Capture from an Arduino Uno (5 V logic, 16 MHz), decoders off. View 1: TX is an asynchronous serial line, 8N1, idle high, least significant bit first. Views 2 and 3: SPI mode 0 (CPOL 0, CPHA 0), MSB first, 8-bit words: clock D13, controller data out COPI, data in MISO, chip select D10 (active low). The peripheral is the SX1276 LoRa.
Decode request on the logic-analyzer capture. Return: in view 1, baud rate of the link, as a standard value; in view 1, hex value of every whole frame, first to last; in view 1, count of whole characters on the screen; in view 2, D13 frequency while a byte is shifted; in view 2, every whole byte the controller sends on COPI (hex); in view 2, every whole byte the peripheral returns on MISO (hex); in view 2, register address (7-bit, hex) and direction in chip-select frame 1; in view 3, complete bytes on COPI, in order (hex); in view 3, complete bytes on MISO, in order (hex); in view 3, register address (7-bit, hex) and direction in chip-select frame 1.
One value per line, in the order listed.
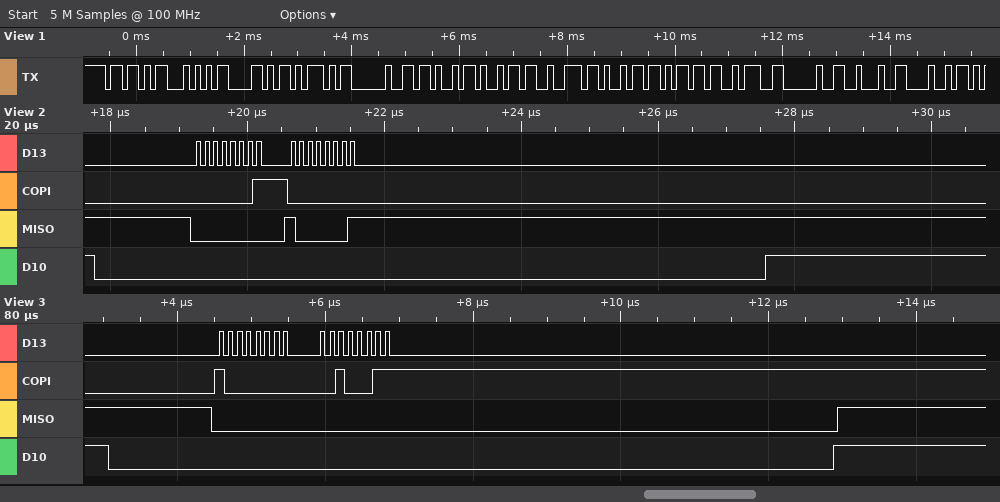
9600 baud
5B 54 58 5D 20 4B 69 72 69 6D 3A 20 22 48
14
8 MHz
0x01 0x00
0x00 0x81
0x01 read
80 23
00 00
0x00 write
